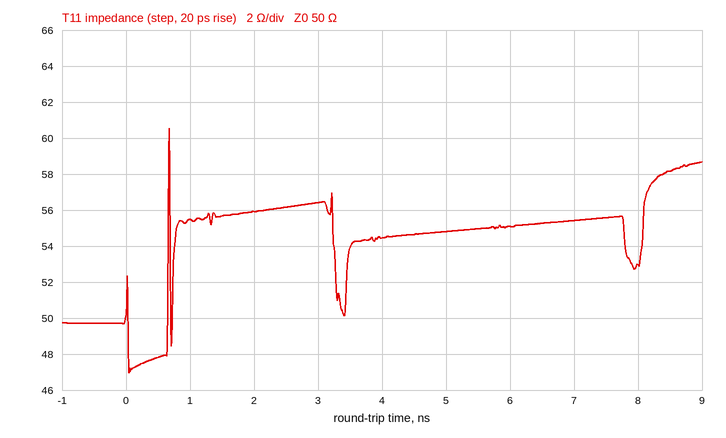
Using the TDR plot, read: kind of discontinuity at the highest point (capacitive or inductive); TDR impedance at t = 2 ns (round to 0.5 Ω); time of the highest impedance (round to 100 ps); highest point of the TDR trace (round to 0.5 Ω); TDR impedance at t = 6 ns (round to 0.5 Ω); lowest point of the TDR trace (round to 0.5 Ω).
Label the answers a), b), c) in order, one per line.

a) inductive
b) 56.0 Ω
c) 700 ps
d) 60.5 Ω
e) 55.0 Ω
f) 47.0 Ω
